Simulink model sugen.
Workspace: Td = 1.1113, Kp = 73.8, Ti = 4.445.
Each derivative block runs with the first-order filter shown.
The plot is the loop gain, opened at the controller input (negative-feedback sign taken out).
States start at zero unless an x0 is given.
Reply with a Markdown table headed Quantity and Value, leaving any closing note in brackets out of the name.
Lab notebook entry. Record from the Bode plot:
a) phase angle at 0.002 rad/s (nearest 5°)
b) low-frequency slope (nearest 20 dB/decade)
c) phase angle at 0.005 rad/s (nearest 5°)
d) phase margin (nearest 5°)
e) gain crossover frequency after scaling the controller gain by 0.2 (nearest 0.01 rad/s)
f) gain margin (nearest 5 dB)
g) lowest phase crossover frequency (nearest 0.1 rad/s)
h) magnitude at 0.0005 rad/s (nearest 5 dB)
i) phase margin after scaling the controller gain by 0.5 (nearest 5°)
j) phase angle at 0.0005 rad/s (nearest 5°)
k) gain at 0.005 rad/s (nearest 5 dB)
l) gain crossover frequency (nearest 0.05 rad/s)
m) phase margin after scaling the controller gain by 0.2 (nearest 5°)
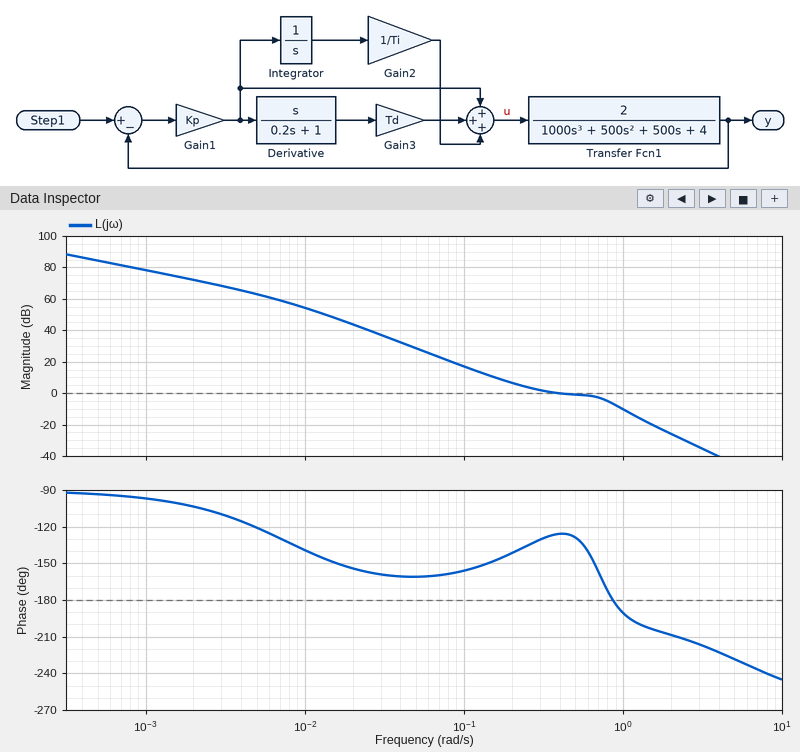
| Quantity | Value |
|---|---|
| phase angle at 0.002 rad/s | -105° |
| low-frequency slope | -20 dB/decade |
| phase angle at 0.005 rad/s | -120° |
| phase margin | 55° |
| gain crossover frequency after scaling the controller gain by 0.2 | 0.12 rad/s |
| gain margin | 5 dB |
| lowest phase crossover frequency | 0.9 rad/s |
| magnitude at 0.0005 rad/s | 85 dB |
| phase margin after scaling the controller gain by 0.5 | 40° |
| phase angle at 0.0005 rad/s | -95° |
| gain at 0.005 rad/s | 65 dB |
| gain crossover frequency | 0.40 rad/s |
| phase margin after scaling the controller gain by 0.2 | 25° |
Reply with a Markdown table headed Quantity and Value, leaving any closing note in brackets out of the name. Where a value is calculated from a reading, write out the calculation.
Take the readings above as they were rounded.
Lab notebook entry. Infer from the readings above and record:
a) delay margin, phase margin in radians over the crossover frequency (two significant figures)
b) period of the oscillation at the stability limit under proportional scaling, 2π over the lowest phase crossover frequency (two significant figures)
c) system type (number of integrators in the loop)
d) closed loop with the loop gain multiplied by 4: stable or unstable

| Quantity | Value |
|---|---|
| delay margin, phase margin in radians over the crossover frequency | 55 × π / 180 / 0.4 = 2.4 s |
| period of the oscillation at the stability limit under proportional scaling, 2π over the lowest phase crossover frequency | 2π / 0.9 = 7.0 s |
| system type | 1 |
| closed loop with the loop gain multiplied by 4: stable or unstable | unstable |
